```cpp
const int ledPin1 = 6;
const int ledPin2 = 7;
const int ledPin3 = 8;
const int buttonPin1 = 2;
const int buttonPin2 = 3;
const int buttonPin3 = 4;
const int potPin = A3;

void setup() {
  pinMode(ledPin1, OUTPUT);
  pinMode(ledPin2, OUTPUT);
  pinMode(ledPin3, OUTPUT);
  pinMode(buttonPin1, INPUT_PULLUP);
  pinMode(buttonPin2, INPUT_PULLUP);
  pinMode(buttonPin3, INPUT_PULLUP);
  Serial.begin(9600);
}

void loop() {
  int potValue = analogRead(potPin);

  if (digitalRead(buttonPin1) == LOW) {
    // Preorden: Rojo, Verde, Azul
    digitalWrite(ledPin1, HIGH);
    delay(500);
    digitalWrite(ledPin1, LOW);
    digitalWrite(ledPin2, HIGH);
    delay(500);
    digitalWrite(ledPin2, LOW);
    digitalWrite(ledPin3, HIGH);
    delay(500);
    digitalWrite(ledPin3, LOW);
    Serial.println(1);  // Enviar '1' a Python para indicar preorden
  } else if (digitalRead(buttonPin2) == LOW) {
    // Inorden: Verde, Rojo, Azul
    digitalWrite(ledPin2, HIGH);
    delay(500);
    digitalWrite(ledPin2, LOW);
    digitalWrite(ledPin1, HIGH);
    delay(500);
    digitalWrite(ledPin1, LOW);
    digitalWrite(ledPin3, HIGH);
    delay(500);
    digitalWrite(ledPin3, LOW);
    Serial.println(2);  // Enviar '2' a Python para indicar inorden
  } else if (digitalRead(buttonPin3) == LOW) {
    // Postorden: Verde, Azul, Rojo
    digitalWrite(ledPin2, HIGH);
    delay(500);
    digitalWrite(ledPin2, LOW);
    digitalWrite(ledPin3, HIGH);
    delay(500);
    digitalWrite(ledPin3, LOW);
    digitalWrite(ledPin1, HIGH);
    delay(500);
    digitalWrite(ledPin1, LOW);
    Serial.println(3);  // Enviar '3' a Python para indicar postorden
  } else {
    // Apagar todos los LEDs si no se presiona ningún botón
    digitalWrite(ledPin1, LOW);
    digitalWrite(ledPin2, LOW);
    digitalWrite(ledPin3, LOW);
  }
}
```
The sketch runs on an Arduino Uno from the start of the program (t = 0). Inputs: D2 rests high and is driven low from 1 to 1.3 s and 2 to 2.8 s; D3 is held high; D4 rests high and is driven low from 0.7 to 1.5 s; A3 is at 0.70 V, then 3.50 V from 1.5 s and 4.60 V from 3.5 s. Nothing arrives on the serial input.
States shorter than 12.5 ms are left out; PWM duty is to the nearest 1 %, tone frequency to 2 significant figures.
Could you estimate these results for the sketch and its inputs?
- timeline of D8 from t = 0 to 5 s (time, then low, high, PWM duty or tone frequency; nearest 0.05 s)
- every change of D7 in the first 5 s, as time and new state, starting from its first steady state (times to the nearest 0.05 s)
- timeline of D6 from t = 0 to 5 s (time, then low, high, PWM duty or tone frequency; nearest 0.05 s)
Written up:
0 s low; 1.2 s high; 1.7 s low; 3.2 s high; 3.7 s low
0 s low; 0.7 s high; 1.2 s low; 2.7 s high; 3.2 s low
0 s low; 1.7 s high; 2.7 s low
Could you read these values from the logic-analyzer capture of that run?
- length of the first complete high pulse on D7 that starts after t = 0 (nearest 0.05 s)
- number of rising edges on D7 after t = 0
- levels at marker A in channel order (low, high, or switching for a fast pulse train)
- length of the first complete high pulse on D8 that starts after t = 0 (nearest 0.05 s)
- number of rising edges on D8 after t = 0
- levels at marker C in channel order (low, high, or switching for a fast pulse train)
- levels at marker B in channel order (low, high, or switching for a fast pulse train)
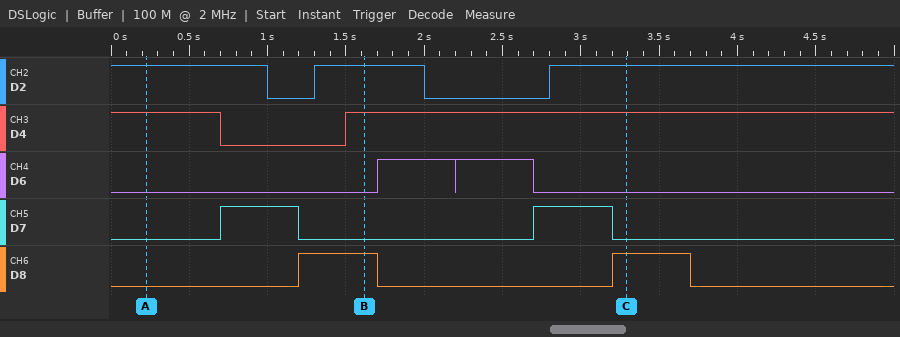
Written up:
0.50 s
2
D2 high, D4 high, D6 low, D7 low, D8 low
0.50 s
2
D2 high, D4 high, D6 low, D7 low, D8 high
D2 high, D4 high, D6 low, D7 low, D8 high
